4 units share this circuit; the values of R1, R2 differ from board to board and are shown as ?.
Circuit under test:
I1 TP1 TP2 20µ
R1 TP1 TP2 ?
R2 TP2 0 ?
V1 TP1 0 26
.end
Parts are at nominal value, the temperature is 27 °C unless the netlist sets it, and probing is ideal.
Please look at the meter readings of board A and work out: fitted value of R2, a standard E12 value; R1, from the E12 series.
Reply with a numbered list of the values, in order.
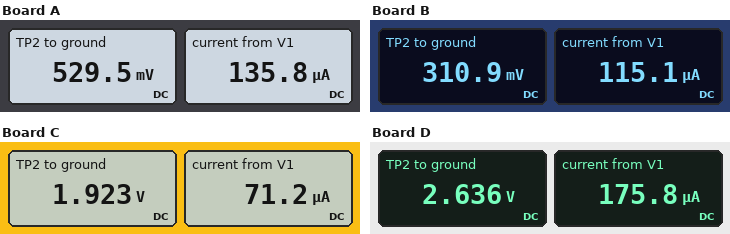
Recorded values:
1. 3.9 kΩ
2. 220 kΩ
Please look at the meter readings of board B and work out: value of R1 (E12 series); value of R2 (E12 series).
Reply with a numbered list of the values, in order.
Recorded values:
1. 270 kΩ
2. 2.7 kΩ
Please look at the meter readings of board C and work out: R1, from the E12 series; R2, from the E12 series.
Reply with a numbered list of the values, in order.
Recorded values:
1. 470 kΩ
2. 27 kΩ
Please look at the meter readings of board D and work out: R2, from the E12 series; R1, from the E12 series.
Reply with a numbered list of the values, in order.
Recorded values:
1. 15 kΩ
2. 150 kΩ
